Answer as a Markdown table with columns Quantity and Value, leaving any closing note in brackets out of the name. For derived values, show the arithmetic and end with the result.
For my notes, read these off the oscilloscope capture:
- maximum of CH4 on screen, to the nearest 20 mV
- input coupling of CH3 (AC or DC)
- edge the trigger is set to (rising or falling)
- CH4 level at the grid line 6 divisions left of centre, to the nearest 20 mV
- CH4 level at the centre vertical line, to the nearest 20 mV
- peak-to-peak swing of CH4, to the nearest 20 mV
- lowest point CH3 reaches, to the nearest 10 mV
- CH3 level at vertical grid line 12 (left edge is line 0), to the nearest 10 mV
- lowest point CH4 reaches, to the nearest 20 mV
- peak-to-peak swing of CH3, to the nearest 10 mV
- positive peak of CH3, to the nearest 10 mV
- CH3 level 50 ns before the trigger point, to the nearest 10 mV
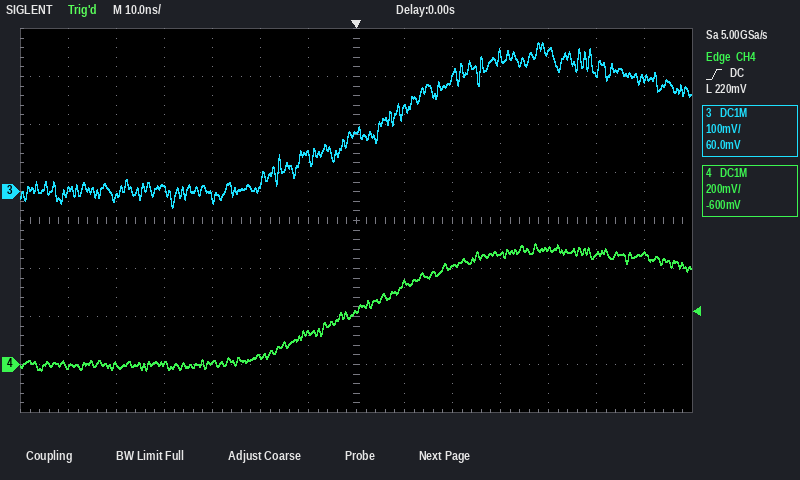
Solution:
| Quantity | Value |
|---|---|
| maximum of CH4 on screen, to the nearest 20 mV | 500 mV |
| input coupling of CH3 | DC |
| edge the trigger is set to | rising |
| CH4 level at the grid line 6 divisions left of centre, to the nearest 20 mV | 0 mV |
| CH4 level at the centre vertical line, to the nearest 20 mV | 220 mV |
| peak-to-peak swing of CH4, to the nearest 20 mV | 500 mV − (-20 mV) = 520 mV |
| lowest point CH3 reaches, to the nearest 10 mV | -30 mV |
| CH3 level at vertical grid line 12 (left edge is line 0), to the nearest 10 mV | 250 mV |
| lowest point CH4 reaches, to the nearest 20 mV | -20 mV |
| peak-to-peak swing of CH3, to the nearest 10 mV | 310 mV − (-30 mV) = 340 mV |
| positive peak of CH3, to the nearest 10 mV | 310 mV |
| CH3 level 50 ns before the trigger point, to the nearest 10 mV | -10 mV |
